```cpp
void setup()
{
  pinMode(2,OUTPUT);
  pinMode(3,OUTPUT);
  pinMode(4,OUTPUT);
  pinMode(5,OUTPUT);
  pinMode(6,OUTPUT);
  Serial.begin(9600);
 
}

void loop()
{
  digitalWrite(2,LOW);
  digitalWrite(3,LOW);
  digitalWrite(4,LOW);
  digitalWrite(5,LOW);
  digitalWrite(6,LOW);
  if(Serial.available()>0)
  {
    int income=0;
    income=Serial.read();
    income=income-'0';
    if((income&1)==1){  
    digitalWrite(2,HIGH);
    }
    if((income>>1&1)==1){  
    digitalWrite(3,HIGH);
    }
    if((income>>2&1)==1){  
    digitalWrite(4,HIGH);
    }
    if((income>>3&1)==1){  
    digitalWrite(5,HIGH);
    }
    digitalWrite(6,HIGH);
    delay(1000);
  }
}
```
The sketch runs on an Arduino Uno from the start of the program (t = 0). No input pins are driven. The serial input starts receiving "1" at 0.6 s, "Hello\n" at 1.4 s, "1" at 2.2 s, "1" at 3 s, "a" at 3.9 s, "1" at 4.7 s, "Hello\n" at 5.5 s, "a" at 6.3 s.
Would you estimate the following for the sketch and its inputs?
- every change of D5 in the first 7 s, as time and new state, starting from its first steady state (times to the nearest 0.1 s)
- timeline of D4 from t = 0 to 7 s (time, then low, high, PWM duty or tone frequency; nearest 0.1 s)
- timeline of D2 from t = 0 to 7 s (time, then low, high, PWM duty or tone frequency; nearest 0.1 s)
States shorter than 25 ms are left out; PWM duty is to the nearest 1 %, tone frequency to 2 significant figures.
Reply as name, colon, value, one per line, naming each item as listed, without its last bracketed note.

every change of D5 in the first 7 s, as time and new state, starting from its first steady state: 0 s low; 1.6 s high; 2.6 s low; 3.6 s high
timeline of D4 from t = 0 to 7 s: 0 s low; 2.6 s high; 6.6 s low
timeline of D2 from t = 0 to 7 s: 0 s low; 0.6 s high; 1.6 s low; 2.6 s high; 3.6 s low; 5.6 s high; 6.6 s low
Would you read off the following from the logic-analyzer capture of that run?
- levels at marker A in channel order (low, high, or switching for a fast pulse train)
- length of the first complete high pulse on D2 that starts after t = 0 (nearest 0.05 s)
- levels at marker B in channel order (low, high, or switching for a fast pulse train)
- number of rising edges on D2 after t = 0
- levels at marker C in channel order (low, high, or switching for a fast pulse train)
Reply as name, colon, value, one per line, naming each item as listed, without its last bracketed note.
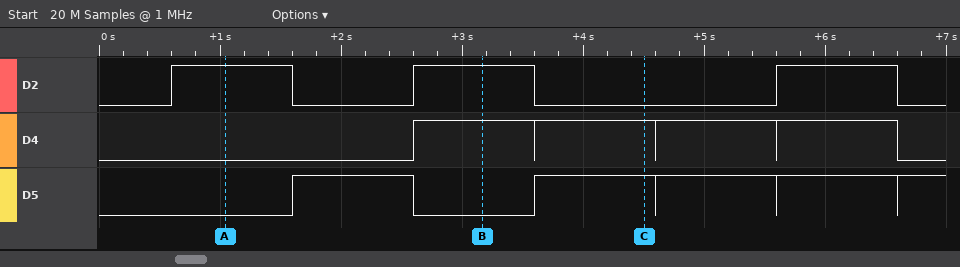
levels at marker A in channel order: D2 high, D4 low, D5 low
length of the first complete high pulse on D2 that starts after t = 0: 1.00 s
levels at marker B in channel order: D2 high, D4 high, D5 low
number of rising edges on D2 after t = 0: 3
levels at marker C in channel order: D2 low, D4 high, D5 high
